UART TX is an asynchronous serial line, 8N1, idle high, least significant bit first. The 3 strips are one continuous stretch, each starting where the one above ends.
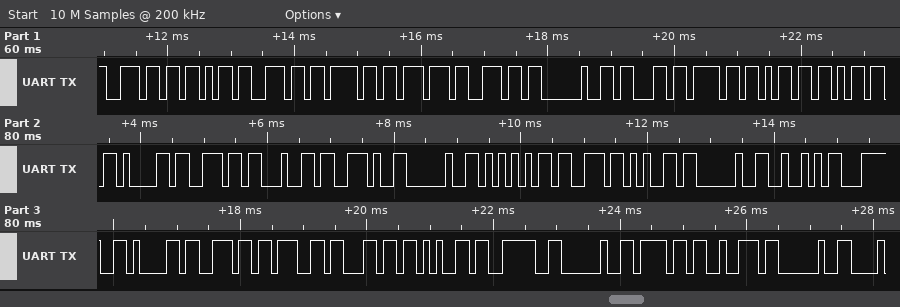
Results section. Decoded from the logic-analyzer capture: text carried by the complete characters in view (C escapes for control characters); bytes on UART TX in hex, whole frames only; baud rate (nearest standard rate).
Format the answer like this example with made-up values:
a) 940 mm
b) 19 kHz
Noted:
a) "nknown command. Use R<angle> or "
b) 6E 6B 6E 6F 77 6E 20 63 6F 6D 6D 61 6E 64 2E 20 55 73 65 20 52 3C 61 6E 67 6C 65 3E 20 6F 72 20
c) 9600 baud
